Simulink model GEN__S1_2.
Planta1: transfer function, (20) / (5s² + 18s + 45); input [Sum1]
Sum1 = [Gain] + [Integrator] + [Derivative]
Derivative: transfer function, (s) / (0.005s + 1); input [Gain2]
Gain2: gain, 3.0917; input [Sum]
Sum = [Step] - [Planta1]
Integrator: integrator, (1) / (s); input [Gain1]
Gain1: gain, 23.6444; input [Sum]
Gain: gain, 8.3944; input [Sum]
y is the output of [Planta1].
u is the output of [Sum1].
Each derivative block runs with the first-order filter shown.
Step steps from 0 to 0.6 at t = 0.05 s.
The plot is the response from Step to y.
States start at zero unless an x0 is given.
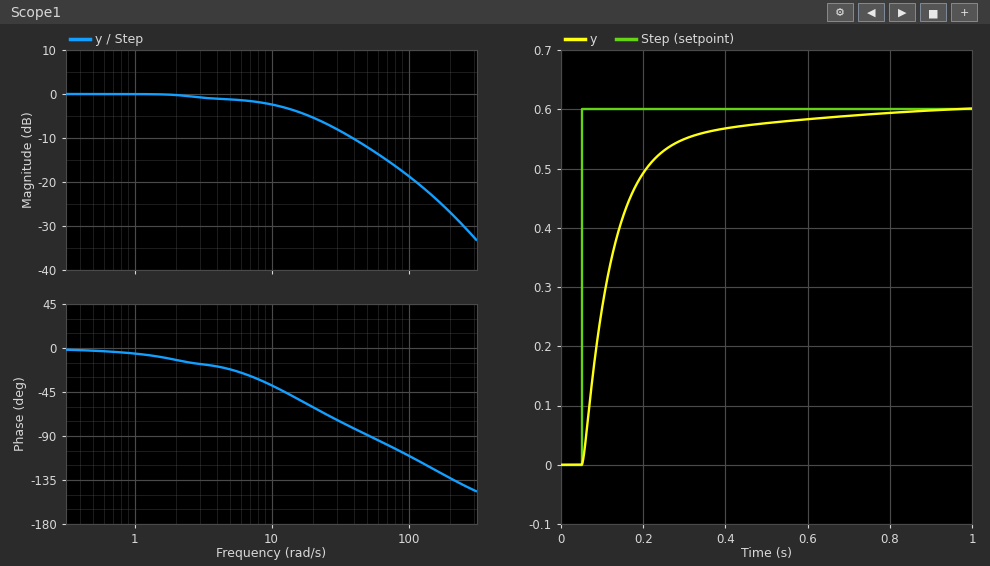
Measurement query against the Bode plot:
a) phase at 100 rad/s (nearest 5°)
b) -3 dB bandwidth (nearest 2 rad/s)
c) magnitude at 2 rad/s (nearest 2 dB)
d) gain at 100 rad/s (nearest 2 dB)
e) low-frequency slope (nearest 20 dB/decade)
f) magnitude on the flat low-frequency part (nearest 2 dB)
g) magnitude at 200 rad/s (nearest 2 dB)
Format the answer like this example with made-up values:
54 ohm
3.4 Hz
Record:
-110°
12 rad/s
0 dB
-18 dB
0 dB/decade
0 dB
-26 dB
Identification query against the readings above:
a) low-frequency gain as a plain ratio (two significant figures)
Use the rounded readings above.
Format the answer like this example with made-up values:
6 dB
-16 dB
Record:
1.0
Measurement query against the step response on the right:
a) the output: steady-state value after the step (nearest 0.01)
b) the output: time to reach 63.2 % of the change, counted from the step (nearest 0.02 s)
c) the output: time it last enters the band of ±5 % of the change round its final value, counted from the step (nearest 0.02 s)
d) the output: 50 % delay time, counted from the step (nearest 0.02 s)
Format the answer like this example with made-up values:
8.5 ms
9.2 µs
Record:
0.60
0.08 s
0.38 s
0.06 s
